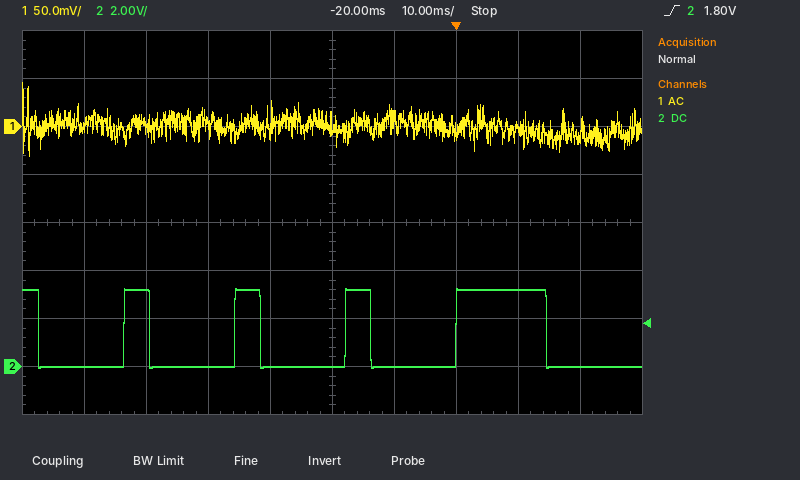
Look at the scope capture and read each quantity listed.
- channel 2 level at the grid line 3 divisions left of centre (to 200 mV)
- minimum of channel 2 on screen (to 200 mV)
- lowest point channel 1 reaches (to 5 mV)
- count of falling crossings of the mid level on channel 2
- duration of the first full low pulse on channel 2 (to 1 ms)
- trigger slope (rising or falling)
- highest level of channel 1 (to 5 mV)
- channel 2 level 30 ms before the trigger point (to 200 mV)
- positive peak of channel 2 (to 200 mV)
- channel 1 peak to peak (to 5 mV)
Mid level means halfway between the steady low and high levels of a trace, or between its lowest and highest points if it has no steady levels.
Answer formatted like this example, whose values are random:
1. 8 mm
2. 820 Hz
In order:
1. 3.2 V
2. 0.0 V
3. -30 mV
4. 5
5. 14 ms
6. rising
7. 45 mV
8. 0.0 V
9. 3.2 V
10. 75 mV
